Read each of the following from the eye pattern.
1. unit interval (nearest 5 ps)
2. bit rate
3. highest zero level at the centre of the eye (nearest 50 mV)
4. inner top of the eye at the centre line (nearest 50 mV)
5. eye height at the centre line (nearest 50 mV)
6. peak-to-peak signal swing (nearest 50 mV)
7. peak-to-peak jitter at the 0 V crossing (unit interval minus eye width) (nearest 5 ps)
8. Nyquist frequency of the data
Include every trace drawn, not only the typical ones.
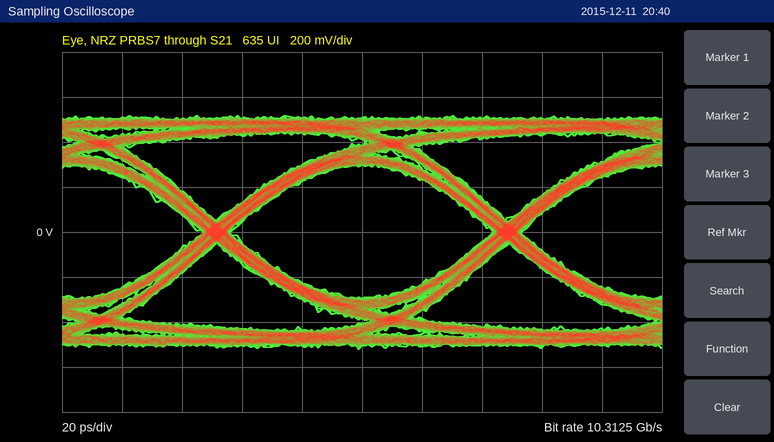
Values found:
95 ps
10.3125 Gb/s
-300 mV
300 mV
600 mV
1.05 V
10 ps
5.15625 GHz
